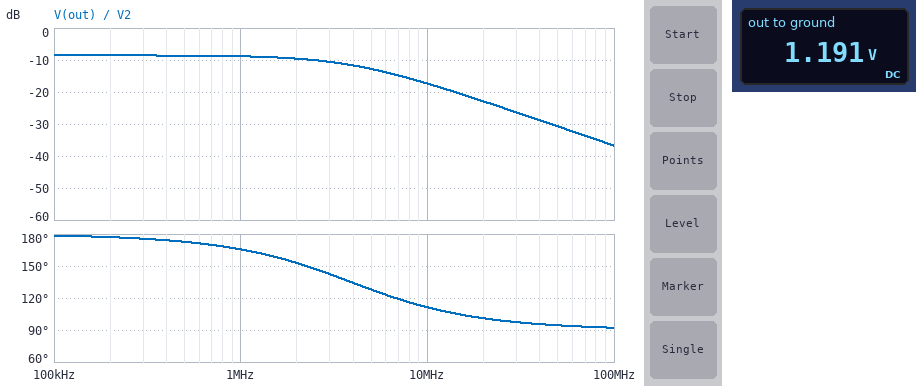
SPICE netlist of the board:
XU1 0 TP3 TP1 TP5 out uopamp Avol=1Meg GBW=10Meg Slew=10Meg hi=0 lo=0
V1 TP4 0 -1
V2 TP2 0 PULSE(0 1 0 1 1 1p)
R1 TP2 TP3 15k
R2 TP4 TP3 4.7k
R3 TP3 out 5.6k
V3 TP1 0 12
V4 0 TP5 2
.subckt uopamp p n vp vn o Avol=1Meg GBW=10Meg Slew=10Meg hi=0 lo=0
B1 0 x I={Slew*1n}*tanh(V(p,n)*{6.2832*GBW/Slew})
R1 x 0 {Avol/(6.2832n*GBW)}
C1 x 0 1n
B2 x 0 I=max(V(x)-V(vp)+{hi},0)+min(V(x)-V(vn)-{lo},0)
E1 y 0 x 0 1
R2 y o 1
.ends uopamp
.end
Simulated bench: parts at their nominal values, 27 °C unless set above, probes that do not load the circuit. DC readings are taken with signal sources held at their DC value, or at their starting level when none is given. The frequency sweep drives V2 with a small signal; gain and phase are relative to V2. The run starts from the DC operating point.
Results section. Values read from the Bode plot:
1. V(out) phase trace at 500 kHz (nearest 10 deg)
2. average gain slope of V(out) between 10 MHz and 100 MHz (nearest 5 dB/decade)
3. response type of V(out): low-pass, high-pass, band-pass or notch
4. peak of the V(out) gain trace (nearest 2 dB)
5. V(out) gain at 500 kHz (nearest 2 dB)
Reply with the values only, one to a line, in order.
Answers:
170 deg
-20 dB/decade
low-pass
-8 dB
-8 dB
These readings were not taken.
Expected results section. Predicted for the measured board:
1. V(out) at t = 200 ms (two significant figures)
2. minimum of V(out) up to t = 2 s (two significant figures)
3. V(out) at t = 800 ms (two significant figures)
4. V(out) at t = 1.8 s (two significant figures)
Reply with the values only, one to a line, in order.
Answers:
1.1 V
820 mV
890 mV
1.1 V
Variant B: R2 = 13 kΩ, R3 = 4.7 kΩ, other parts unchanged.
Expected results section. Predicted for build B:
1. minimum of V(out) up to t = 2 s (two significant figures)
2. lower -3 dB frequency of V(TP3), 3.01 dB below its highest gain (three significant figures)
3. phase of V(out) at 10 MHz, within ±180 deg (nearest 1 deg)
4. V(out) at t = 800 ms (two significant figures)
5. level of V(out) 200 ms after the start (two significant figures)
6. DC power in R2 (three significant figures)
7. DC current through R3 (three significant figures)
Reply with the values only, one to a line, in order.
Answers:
48 mV
5.97 MHz
121 deg
110 mV
300 mV
76.9 µW
76.9 µA
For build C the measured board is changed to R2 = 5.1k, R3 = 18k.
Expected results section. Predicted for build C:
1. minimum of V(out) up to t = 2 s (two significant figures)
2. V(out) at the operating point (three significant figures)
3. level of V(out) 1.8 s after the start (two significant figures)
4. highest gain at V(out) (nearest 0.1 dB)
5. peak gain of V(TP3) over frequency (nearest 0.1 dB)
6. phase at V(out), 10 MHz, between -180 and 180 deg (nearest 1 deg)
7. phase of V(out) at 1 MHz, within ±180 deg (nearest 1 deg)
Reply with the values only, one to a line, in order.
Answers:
2.3 V
3.53 V
3.3 V
1.6 dB
-13.6 dB
100 deg
150 deg
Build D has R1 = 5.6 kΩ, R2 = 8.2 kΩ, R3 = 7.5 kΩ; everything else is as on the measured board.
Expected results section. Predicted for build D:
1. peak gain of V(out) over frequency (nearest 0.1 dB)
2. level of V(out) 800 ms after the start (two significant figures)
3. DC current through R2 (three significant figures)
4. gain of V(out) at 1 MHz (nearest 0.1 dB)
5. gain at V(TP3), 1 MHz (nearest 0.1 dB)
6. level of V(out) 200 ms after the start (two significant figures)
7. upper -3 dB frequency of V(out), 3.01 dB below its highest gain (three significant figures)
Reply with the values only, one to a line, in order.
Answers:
2.5 dB
-160 mV
122 µA
2.1 dB
-17.9 dB
650 mV
3.07 MHz
